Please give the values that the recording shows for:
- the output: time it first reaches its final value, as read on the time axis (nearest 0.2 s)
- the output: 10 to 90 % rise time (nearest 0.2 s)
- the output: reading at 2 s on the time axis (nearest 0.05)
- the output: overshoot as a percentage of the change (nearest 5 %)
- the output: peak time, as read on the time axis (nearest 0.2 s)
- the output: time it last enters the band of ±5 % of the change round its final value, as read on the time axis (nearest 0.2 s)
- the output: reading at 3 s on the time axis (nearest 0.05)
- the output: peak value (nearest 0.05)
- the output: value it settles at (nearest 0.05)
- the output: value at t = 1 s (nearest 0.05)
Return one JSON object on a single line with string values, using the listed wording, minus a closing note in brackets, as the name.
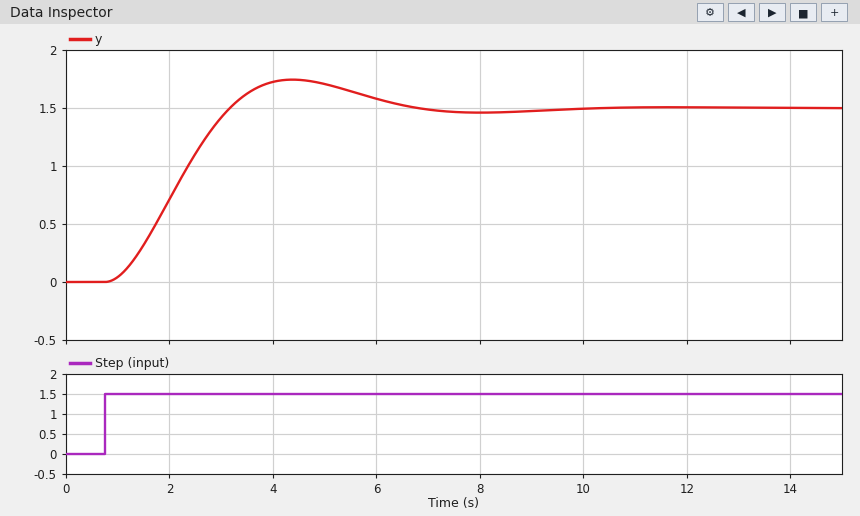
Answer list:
{"the output: time it first reaches its final value, as read on the time axis": "3.2 s", "the output: 10 to 90 % rise time": "1.6 s", "the output: reading at 2 s on the time axis": "0.70", "the output: overshoot as a percentage of the change": "15 %", "the output: peak time, as read on the time axis": "4.4 s", "the output: time it last enters the band of ±5 % of the change round its final value, as read on the time axis": "6.0 s", "the output: reading at 3 s on the time axis": "1.40", "the output: peak value": "1.75", "the output: value it settles at": "1.50", "the output: value at t = 1 s": "0.05"}
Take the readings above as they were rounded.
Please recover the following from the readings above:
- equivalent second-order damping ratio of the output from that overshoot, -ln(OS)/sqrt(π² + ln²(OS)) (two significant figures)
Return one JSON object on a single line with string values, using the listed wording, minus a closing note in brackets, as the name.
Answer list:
{"equivalent second-order damping ratio of the output from that overshoot, -ln(OS)/sqrt(π² + ln²(OS))": "0.52"}
